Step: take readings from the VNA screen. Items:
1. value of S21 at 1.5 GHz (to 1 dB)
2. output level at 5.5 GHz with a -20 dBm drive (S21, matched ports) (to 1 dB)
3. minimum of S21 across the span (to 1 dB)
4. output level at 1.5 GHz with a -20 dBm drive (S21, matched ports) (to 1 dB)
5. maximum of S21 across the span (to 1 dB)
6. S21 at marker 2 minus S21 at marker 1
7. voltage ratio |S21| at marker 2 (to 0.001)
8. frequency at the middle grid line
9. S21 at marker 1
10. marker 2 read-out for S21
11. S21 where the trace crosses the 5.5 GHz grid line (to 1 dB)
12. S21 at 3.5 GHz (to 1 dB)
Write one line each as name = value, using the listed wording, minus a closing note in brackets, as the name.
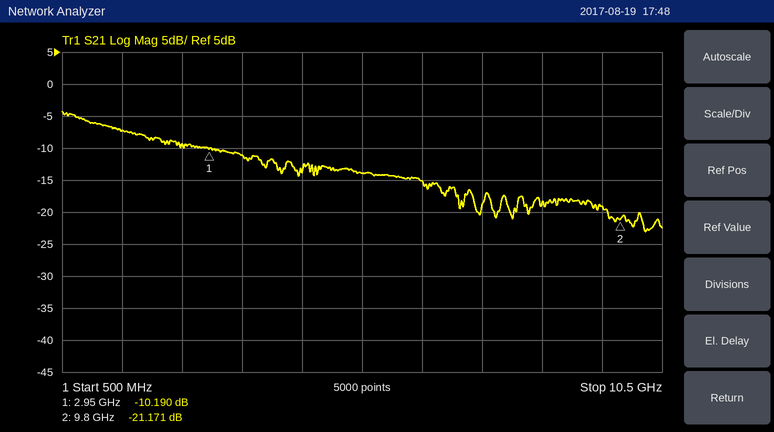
value of S21 at 1.5 GHz = -7 dB
output level at 5.5 GHz with a -20 dBm drive (S21, matched ports) = -34 dBm
minimum of S21 across the span = -23 dB
output level at 1.5 GHz with a -20 dBm drive (S21, matched ports) = -27 dBm
maximum of S21 across the span = -4 dB
S21 at marker 2 minus S21 at marker 1 = -10.981 dB
voltage ratio |S21| at marker 2 = 0.087
frequency at the middle grid line = 5.5 GHz
S21 at marker 1 = -10.190 dB
marker 2 read-out for S21 = -21.171 dB
S21 where the trace crosses the 5.5 GHz grid line = -14 dB
S21 at 3.5 GHz = -11 dB
